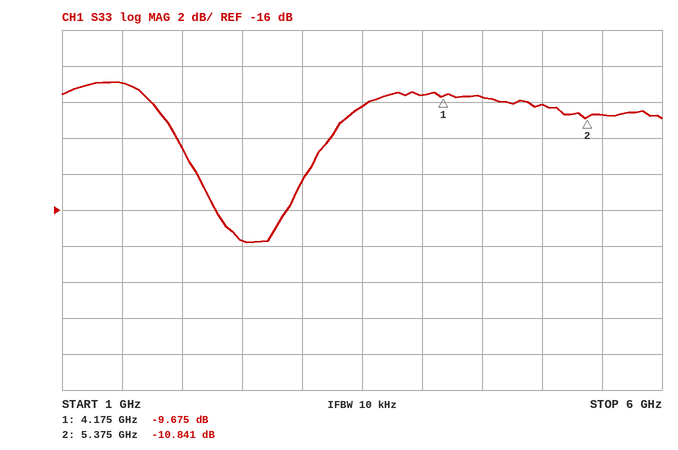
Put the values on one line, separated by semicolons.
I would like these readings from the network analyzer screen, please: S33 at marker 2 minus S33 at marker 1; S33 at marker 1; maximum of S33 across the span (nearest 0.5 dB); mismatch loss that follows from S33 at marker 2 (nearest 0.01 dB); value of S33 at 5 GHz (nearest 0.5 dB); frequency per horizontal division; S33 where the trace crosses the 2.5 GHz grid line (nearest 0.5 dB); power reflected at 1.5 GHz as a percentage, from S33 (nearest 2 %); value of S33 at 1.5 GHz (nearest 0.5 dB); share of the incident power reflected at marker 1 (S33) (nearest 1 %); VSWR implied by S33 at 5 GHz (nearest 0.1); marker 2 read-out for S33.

-1.166 dB; -9.675 dB; -9.0 dB; 0.37 dB; -10.0 dB; 500 MHz; -17.5 dB; 12 %; -9.0 dB; 11 %; 1.9; -10.841 dB
